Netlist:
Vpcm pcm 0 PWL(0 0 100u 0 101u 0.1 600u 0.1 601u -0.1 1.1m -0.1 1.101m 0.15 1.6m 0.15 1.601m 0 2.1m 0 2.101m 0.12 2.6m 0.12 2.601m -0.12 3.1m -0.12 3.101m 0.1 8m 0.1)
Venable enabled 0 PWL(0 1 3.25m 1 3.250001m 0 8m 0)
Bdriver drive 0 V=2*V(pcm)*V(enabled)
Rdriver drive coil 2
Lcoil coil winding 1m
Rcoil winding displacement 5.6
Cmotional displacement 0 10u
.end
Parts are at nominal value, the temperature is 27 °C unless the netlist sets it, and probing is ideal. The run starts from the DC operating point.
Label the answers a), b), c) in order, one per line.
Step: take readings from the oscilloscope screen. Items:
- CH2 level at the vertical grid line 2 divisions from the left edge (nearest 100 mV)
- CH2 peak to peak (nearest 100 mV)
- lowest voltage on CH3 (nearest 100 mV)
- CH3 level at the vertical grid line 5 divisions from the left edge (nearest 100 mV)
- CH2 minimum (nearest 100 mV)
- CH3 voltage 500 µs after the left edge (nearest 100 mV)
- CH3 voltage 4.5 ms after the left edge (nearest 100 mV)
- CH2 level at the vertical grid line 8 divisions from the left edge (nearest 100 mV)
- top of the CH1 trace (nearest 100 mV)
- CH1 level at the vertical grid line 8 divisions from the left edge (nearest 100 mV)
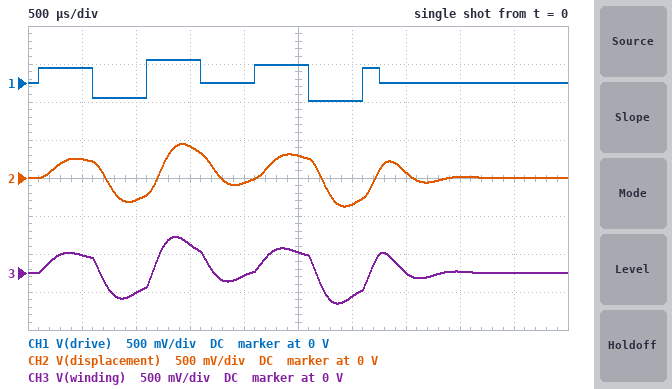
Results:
a) -300 mV
b) 800 mV
c) -400 mV
d) 300 mV
e) -400 mV
f) 200 mV
g) 0 V
h) 0 V
i) 300 mV
j) 0 V
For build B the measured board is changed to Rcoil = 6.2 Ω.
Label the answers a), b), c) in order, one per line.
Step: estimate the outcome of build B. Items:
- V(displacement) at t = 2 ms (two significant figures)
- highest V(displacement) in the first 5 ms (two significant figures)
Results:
a) -63 mV
b) 430 mV
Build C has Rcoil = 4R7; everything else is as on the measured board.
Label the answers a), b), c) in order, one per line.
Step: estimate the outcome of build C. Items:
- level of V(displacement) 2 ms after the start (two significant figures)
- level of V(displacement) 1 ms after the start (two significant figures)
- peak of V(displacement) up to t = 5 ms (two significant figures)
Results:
a) -69 mV
b) -300 mV
c) 470 mV
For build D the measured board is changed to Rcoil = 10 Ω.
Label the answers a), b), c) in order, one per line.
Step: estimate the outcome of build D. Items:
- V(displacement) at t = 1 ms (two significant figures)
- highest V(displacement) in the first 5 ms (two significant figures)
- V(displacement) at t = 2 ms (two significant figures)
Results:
a) -240 mV
b) 350 mV
c) -31 mV
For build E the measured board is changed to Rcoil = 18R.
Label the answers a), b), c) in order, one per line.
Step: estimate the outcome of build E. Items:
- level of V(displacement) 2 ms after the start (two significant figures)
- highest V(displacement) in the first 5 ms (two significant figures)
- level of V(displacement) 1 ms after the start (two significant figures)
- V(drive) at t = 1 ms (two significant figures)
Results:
a) 27 mV
b) 280 mV
c) -160 mV
d) -200 mV
